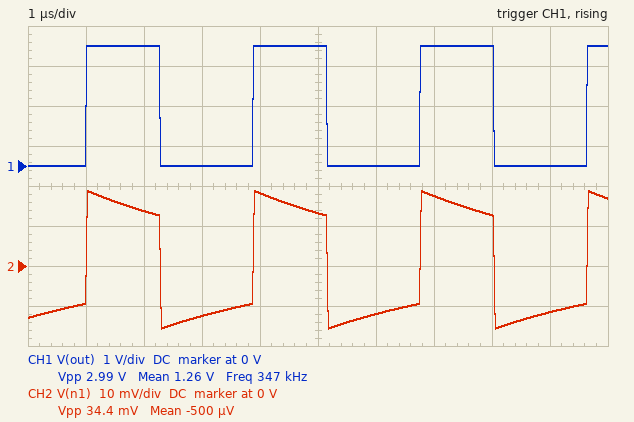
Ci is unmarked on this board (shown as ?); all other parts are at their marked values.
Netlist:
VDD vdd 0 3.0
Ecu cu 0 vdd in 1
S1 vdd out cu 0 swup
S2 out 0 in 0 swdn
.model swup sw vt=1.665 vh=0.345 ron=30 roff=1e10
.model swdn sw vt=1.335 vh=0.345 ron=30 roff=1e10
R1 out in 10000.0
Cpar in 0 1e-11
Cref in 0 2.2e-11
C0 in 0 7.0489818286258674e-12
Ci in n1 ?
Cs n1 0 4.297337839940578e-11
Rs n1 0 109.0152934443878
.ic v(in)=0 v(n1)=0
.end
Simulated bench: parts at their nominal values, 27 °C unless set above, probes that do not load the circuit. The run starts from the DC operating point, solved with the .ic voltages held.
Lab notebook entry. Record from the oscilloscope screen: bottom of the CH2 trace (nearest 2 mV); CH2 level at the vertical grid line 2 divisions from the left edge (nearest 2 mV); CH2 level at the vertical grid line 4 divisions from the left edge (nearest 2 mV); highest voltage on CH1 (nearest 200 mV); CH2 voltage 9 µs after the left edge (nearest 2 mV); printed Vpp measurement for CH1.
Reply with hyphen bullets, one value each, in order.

- -16 mV
- 14 mV
- 18 mV
- 3.0 V
- -12 mV
- 2.99 V
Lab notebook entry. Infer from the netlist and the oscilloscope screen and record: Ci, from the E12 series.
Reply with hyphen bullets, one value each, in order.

- 270 pF
